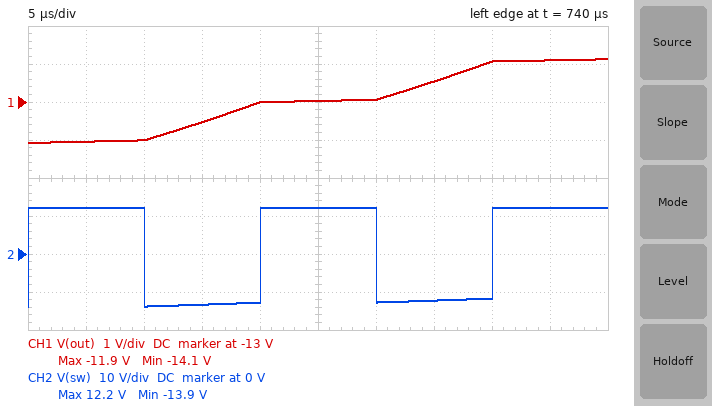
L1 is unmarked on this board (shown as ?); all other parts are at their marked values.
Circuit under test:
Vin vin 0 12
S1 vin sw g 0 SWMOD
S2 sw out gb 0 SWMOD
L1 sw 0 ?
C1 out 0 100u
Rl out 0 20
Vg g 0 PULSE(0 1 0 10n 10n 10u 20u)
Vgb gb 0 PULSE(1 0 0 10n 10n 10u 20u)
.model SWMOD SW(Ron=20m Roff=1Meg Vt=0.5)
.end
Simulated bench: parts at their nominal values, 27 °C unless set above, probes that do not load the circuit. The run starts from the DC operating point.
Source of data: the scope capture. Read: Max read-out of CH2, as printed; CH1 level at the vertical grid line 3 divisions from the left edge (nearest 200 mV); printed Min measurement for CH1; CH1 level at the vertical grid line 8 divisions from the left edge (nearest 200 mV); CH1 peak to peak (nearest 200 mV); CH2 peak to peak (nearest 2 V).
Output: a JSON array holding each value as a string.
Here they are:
["12.2 V", "-13.6 V", "-14.1 V", "-12.0 V", "2.2 V", "26 V"]
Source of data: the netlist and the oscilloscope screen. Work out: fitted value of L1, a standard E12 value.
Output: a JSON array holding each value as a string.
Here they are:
["68 µH"]
